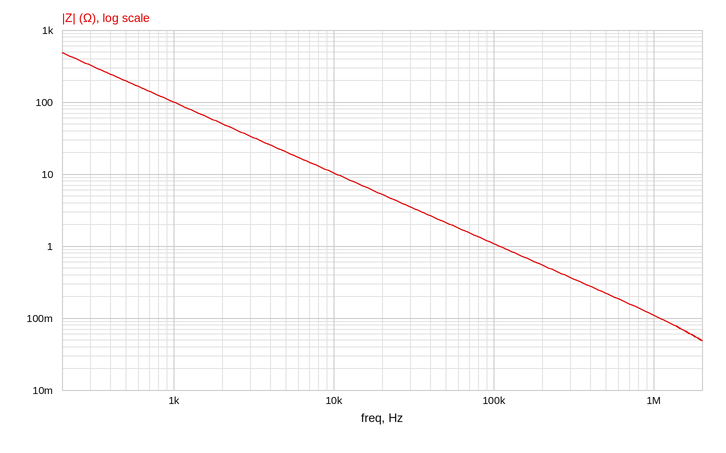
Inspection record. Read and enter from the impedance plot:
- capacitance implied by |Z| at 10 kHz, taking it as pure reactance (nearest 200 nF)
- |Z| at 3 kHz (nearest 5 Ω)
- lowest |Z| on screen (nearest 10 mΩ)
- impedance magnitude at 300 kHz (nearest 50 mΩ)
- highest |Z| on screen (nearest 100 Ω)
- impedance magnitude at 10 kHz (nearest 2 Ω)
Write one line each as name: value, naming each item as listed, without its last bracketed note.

capacitance implied by |Z| at 10 kHz, taking it as pure reactance: 1.6 µF
|Z| at 3 kHz: 35 Ω
lowest |Z| on screen: 50 mΩ
impedance magnitude at 300 kHz: 350 mΩ
highest |Z| on screen: 500 Ω
impedance magnitude at 10 kHz: 10 Ω
